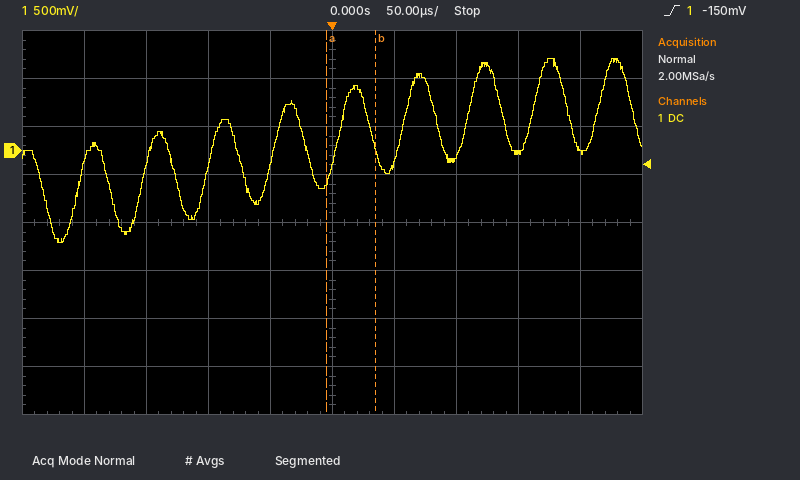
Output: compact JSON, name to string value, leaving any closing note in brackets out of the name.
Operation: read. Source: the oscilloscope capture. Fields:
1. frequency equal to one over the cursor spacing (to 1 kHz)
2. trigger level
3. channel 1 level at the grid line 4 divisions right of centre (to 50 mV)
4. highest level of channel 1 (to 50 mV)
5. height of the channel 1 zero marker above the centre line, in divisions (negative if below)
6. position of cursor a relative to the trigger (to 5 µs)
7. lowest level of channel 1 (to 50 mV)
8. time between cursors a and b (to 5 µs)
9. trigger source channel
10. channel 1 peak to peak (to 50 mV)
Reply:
{"frequency equal to one over the cursor spacing": "25 kHz", "trigger level": "-150 mV", "channel 1 level at the grid line 4 divisions right of centre": "0 mV", "highest level of channel 1": "950 mV", "height of the channel 1 zero marker above the centre line, in divisions": "+1.5 div", "position of cursor a relative to the trigger": "-5 µs", "lowest level of channel 1": "-950 mV", "time between cursors a and b": "40 µs", "trigger source channel": "channel 1", "channel 1 peak to peak": "1.90 V"}
